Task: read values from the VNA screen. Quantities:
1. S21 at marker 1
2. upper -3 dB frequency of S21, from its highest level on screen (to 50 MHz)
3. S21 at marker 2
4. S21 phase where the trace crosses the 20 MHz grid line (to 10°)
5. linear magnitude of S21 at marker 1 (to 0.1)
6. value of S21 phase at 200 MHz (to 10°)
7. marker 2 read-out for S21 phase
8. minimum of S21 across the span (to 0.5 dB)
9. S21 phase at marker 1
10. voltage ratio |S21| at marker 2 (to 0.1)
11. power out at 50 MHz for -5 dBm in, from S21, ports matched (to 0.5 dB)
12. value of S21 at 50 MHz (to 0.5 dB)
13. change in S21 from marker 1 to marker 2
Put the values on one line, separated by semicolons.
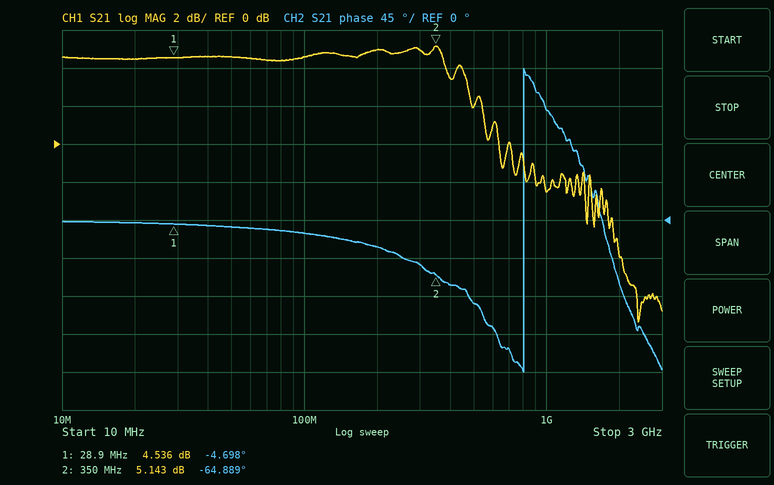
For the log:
4.536 dB; 500 MHz; 5.143 dB; 0°; 1.7; -30°; -64.889°; -9.5 dB; -4.698°; 1.8; -0.5 dBm; 4.5 dB; 0.607 dB
